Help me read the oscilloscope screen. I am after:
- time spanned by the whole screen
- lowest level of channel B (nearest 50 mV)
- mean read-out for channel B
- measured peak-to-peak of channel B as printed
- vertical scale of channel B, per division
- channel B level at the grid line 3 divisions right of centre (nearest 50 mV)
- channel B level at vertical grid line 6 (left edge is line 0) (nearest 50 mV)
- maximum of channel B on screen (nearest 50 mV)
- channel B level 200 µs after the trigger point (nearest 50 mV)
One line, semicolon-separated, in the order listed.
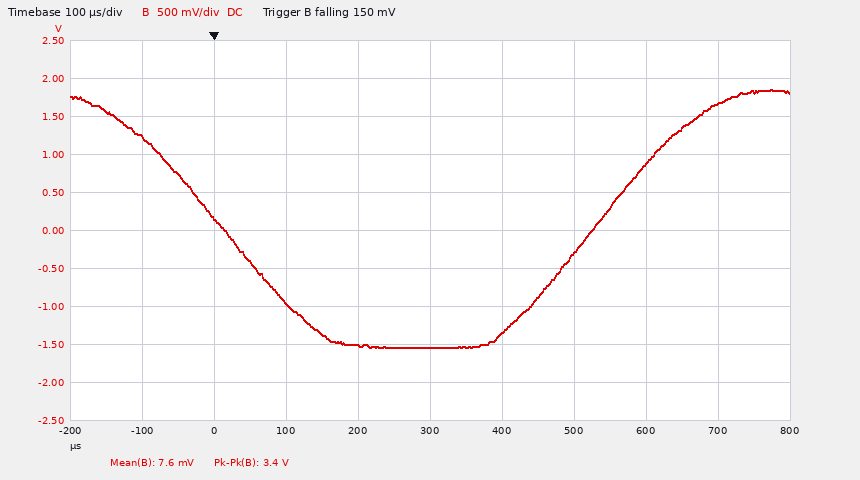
1 ms; -1.55 V; 7.6 mV; 3.4 V; 500 mV; 900 mV; -1.35 V; 1.85 V; -1.50 V
